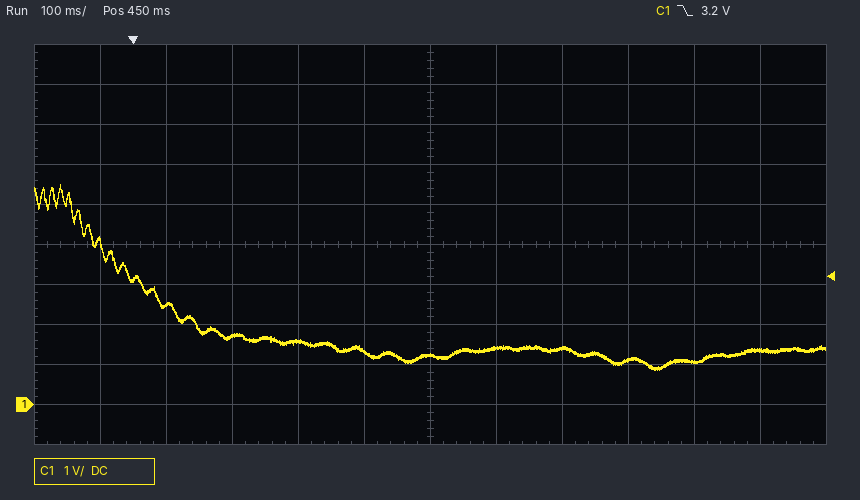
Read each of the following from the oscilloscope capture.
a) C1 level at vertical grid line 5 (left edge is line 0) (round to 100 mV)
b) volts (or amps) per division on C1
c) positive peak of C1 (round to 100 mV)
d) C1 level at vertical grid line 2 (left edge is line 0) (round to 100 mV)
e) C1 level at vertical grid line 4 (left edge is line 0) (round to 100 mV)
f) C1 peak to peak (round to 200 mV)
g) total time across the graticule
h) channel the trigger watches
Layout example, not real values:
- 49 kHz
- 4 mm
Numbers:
- 1.3 V
- 1 V
- 5.5 V
- 2.5 V
- 1.6 V
- 4.6 V
- 1.2 s
- C1
